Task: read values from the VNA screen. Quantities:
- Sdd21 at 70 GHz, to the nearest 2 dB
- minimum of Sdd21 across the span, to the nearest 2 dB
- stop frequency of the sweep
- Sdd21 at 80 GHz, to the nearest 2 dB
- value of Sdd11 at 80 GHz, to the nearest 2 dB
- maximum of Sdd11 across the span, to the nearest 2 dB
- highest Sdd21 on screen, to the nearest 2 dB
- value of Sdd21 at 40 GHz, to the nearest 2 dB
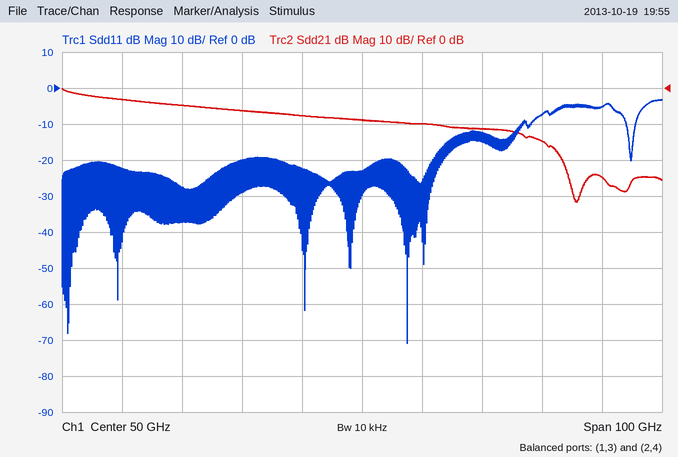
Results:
-12 dB
-32 dB
100 GHz
-14 dB
-8 dB
-4 dB
0 dB
-8 dB
